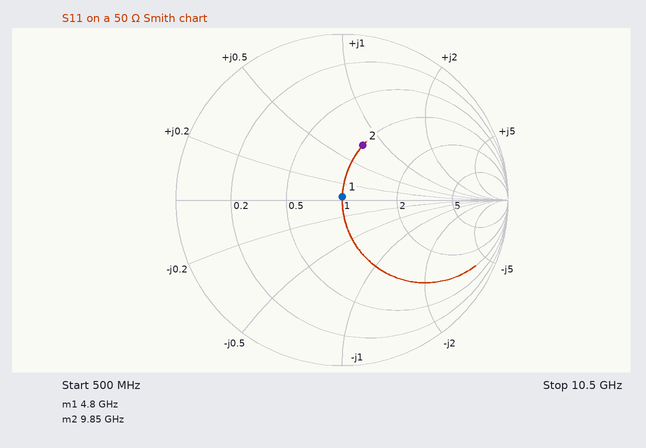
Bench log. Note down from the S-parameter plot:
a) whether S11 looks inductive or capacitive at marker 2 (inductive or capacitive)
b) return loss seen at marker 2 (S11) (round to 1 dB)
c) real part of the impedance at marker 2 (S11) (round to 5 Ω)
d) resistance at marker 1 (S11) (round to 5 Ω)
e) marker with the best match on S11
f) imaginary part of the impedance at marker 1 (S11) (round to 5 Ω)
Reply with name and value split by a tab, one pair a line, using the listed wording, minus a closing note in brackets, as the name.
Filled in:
whether S11 looks inductive or capacitive at marker 2	inductive
return loss seen at marker 2 (S11)	9 dB
real part of the impedance at marker 2 (S11)	50 Ω
resistance at marker 1 (S11)	50 Ω
marker with the best match on S11	marker 1
imaginary part of the impedance at marker 1 (S11)	0 Ω
